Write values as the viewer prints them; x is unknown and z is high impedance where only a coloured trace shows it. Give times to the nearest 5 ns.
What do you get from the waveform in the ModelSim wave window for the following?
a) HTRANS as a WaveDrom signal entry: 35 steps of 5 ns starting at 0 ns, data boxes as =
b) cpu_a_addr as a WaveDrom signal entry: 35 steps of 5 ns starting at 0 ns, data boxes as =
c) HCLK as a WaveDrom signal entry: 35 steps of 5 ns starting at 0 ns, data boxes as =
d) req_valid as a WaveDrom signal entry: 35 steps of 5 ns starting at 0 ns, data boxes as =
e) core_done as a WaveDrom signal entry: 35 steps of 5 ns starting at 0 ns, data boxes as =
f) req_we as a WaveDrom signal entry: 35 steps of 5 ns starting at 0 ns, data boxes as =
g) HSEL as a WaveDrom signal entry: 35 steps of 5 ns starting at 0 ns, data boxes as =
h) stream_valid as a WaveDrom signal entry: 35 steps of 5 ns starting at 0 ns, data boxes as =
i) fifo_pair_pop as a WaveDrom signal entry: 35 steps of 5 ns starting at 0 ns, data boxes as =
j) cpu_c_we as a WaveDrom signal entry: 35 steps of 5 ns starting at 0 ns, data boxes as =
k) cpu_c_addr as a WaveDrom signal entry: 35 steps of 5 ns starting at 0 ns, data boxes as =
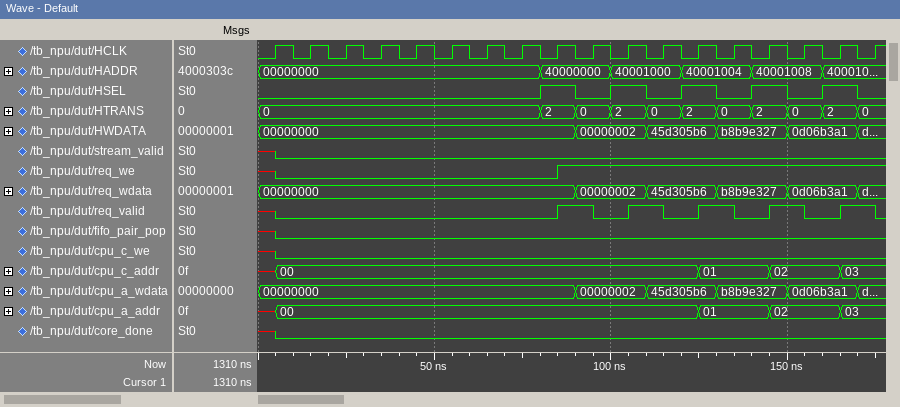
{name: 'HTRANS', wave: '=...............=.=.=.=.=.=.=.=.=.=', data: '0 2 0 2 0 2 0 2 0 2 0'}
{name: 'cpu_a_addr', wave: 'x=.......................=...=...=.', data: '00 01 02 03'}
{name: 'HCLK', wave: '01010101010101010101010101010101010'}
{name: 'req_valid', wave: 'x0...............1.0.1.0.1.0.1.0.1.'}
{name: 'core_done', wave: 'x0.................................'}
{name: 'req_we', wave: 'x0...............1.................'}
{name: 'HSEL', wave: '0...............1.0.1.0.1.0.1.0.1.0'}
{name: 'stream_valid', wave: 'x0.................................'}
{name: 'fifo_pair_pop', wave: 'x0.................................'}
{name: 'cpu_c_we', wave: 'x0.................................'}
{name: 'cpu_c_addr', wave: 'x=.......................=...=...=.', data: '00 01 02 03'}
